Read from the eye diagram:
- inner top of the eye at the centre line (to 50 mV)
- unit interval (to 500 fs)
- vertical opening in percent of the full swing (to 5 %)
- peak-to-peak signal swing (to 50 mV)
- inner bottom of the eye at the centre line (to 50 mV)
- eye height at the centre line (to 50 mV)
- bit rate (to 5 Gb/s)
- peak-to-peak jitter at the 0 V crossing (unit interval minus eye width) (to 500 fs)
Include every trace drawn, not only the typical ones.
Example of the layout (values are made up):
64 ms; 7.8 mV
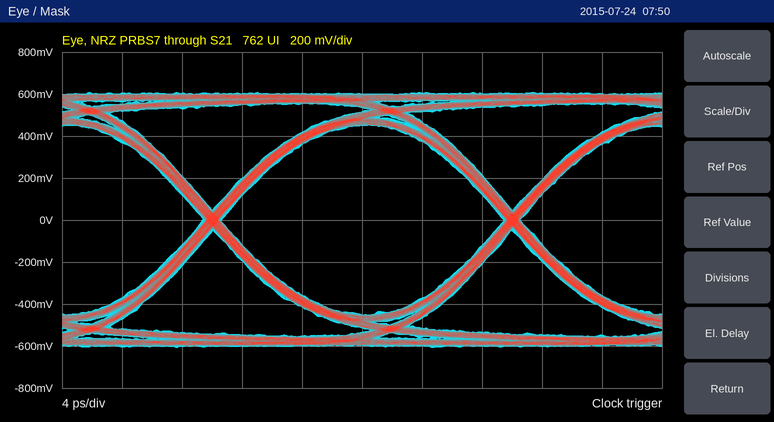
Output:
450 mV; 20.0 ps; 75 %; 1.20 V; -450 mV; 900 mV; 50 Gb/s; 1.0 ps
